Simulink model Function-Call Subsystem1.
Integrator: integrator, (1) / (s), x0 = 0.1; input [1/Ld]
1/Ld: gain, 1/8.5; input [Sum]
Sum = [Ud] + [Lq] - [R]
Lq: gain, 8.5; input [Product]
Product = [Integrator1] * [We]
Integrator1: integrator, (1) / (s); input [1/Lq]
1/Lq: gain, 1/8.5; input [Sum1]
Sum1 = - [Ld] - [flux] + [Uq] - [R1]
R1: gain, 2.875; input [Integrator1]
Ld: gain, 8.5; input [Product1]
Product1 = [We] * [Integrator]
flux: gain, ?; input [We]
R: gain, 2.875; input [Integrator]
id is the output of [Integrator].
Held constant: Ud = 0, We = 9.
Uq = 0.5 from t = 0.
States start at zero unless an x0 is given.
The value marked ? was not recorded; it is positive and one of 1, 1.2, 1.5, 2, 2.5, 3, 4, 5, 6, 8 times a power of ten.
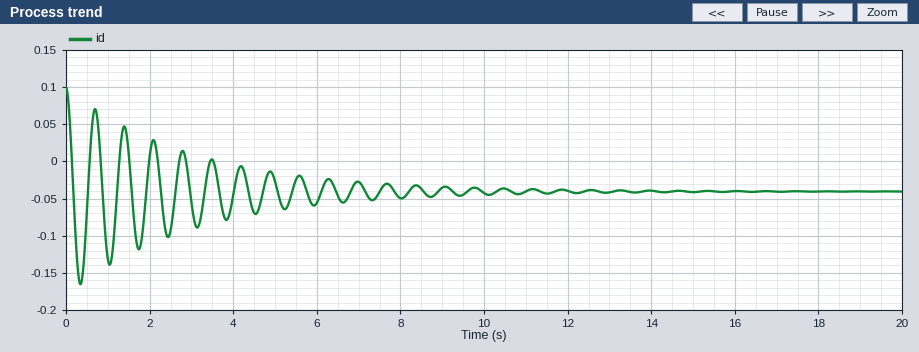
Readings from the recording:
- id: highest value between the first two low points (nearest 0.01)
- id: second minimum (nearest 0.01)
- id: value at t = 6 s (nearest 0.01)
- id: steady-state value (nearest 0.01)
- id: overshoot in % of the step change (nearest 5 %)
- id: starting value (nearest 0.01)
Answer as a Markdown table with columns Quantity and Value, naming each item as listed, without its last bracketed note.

| Quantity | Value |
|---|---|
| id: highest value between the first two low points | 0.07 |
| id: second minimum | -0.14 |
| id: value at t = 6 s | -0.06 |
| id: steady-state value | -0.04 |
| id: overshoot in % of the step change | 90 % |
| id: starting value | 0.10 |
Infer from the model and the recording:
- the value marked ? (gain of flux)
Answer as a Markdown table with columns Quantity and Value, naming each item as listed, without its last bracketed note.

| Quantity | Value |
|---|---|
| the value marked ? | 0.4 |
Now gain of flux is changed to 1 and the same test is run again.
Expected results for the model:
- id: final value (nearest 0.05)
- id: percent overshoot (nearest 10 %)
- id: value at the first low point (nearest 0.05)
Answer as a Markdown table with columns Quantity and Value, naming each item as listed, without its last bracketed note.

| Quantity | Value |
|---|---|
| id: final value | -0.10 |
| id: percent overshoot | 90 % |
| id: value at the first low point | -0.30 |
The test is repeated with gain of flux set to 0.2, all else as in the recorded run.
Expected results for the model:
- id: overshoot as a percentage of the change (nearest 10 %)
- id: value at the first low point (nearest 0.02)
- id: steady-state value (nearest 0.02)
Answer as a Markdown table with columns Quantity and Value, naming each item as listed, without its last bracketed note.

| Quantity | Value |
|---|---|
| id: overshoot as a percentage of the change | 90 % |
| id: value at the first low point | -0.12 |
| id: steady-state value | -0.02 |
